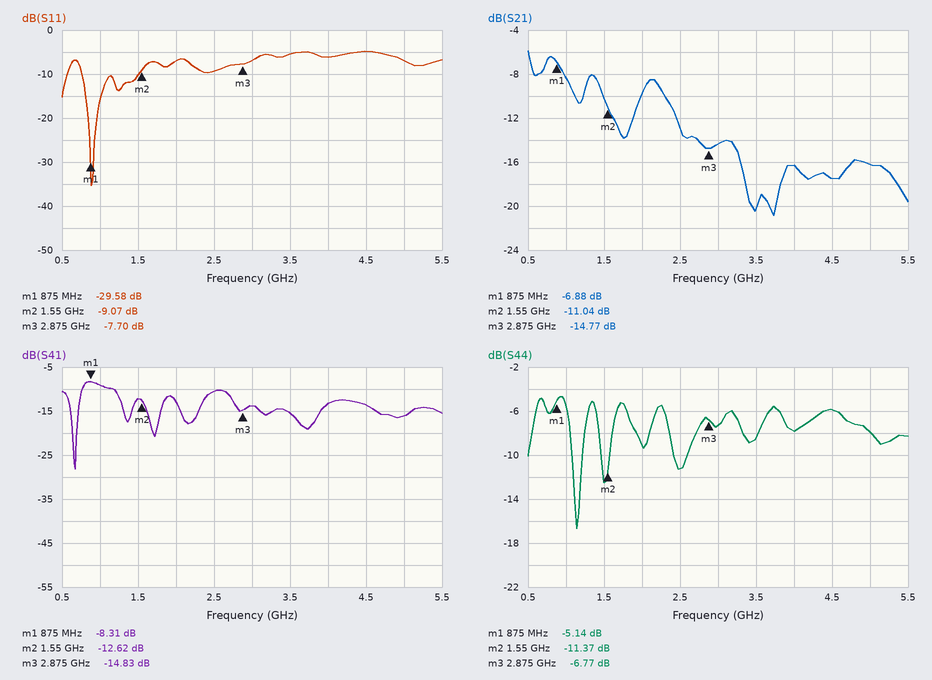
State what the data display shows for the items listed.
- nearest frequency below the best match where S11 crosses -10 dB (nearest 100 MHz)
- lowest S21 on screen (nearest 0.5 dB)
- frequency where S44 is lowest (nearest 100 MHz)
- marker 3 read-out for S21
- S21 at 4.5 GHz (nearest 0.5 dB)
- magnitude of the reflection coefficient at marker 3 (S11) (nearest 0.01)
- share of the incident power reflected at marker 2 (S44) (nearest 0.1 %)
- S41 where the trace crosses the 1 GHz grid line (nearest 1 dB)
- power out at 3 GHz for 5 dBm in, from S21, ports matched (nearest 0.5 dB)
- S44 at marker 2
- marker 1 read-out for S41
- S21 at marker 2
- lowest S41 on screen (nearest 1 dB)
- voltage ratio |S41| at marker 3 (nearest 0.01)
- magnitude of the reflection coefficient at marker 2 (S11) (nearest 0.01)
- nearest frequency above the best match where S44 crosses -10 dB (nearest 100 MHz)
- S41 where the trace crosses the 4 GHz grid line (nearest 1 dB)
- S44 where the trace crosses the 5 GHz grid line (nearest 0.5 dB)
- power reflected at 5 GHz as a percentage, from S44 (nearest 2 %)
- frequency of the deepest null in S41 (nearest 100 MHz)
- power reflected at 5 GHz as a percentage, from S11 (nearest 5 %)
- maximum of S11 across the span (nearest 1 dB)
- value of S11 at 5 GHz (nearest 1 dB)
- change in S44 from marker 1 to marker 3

800 MHz
-21.0 dB
1.1 GHz
-14.77 dB
-17.5 dB
0.41
7.3 %
-9 dB
-9.5 dBm
-11.37 dB
-8.31 dB
-11.04 dB
-28 dB
0.18
0.35
1.2 GHz
-13 dB
-8.0 dB
16 %
700 MHz
20 %
-5 dB
-7 dB
-1.63 dB
